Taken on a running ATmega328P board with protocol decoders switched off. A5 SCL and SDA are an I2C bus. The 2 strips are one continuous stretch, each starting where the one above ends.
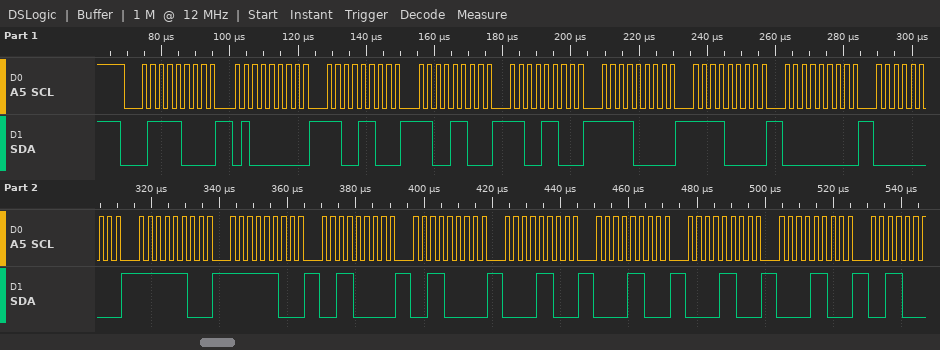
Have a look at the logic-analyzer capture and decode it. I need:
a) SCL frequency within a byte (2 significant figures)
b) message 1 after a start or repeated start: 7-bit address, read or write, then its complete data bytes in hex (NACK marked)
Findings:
400 kHz
0x3C write: 40 CC CC CC F0 F0 00 00 FC FC 30 30 0C 0C 0C 0C
